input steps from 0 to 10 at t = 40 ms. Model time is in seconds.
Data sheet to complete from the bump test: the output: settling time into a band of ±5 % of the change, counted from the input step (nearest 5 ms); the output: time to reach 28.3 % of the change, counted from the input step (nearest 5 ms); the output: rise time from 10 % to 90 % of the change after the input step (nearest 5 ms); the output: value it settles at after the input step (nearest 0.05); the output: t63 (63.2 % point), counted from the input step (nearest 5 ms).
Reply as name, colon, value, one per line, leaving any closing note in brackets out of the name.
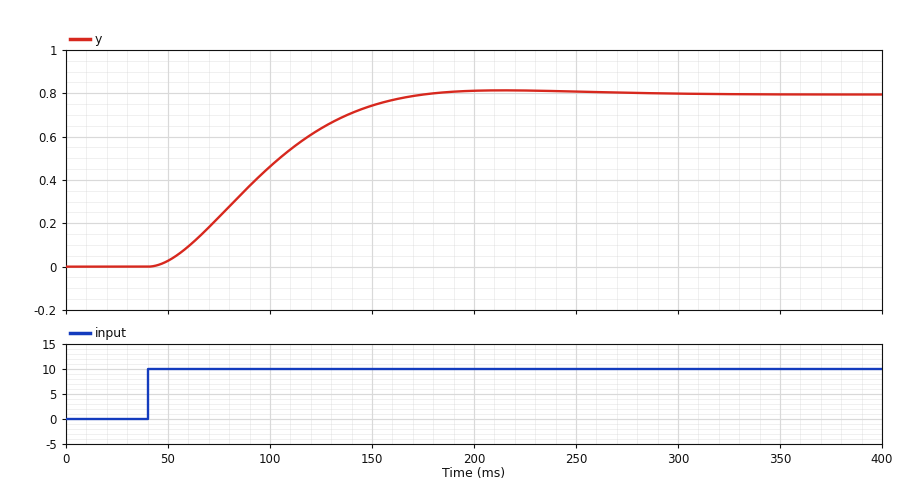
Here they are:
the output: settling time into a band of ±5 % of the change, counted from the input step: 115 ms
the output: time to reach 28.3 % of the change, counted from the input step: 35 ms
the output: rise time from 10 % to 90 % of the change after the input step: 85 ms
the output: value it settles at after the input step: 0.80
the output: t63 (63.2 % point), counted from the input step: 65 ms
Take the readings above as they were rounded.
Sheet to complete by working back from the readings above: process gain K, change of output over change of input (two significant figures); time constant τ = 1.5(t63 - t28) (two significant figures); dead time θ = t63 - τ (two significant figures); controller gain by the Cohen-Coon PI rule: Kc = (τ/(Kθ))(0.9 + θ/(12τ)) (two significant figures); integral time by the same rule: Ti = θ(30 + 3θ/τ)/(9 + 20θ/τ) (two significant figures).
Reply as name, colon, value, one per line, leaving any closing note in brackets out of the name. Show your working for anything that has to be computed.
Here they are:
process gain K, change of output over change of input: (0.8 - 0) / 10 = 0.080
time constant τ = 1.5(t63 - t28): 1.5 × (65 - 35) = 45 ms
dead time θ = t63 - τ: 65 - 45 = 20 ms
controller gain by the Cohen-Coon PI rule: Kc = (τ/(Kθ))(0.9 + θ/(12τ)): 45 / (0.08 × 20) × (0.9 + 20 / (12 × 45)) = 26
integral time by the same rule: Ti = θ(30 + 3θ/τ)/(9 + 20θ/τ): 20 × (30 + 3 × 20 / 45) / (9 + 20 × 20 / 45) = 35 ms
